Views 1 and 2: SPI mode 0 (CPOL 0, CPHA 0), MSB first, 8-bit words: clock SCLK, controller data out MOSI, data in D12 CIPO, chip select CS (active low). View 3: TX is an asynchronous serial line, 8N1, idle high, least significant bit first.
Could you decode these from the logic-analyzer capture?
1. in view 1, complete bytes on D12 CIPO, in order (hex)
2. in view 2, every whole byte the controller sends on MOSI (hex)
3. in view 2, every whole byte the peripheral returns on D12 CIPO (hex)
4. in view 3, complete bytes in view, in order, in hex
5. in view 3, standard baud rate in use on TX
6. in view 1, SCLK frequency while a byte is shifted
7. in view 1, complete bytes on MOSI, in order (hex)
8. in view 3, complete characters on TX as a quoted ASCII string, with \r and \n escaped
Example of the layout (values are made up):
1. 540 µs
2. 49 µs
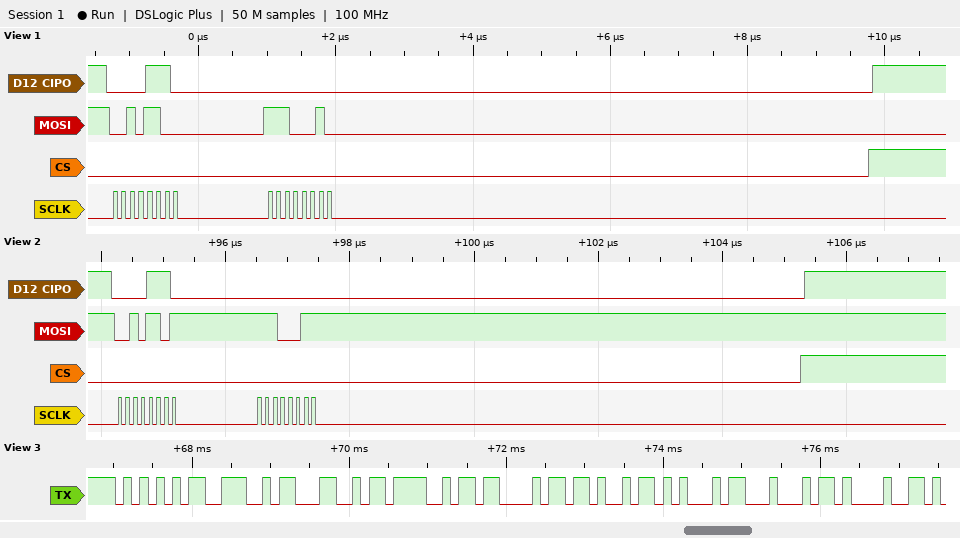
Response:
1. 0x0E 0x00
2. 2D E3
3. 0E 00
4. 0x55 0x4E 0x4C 0x4F 0x43 0x4B 0x45 0x44 0x21
5. 9600 baud
6. 8 MHz
7. 0x2C 0xE2
8. "UNLOCKED!"
